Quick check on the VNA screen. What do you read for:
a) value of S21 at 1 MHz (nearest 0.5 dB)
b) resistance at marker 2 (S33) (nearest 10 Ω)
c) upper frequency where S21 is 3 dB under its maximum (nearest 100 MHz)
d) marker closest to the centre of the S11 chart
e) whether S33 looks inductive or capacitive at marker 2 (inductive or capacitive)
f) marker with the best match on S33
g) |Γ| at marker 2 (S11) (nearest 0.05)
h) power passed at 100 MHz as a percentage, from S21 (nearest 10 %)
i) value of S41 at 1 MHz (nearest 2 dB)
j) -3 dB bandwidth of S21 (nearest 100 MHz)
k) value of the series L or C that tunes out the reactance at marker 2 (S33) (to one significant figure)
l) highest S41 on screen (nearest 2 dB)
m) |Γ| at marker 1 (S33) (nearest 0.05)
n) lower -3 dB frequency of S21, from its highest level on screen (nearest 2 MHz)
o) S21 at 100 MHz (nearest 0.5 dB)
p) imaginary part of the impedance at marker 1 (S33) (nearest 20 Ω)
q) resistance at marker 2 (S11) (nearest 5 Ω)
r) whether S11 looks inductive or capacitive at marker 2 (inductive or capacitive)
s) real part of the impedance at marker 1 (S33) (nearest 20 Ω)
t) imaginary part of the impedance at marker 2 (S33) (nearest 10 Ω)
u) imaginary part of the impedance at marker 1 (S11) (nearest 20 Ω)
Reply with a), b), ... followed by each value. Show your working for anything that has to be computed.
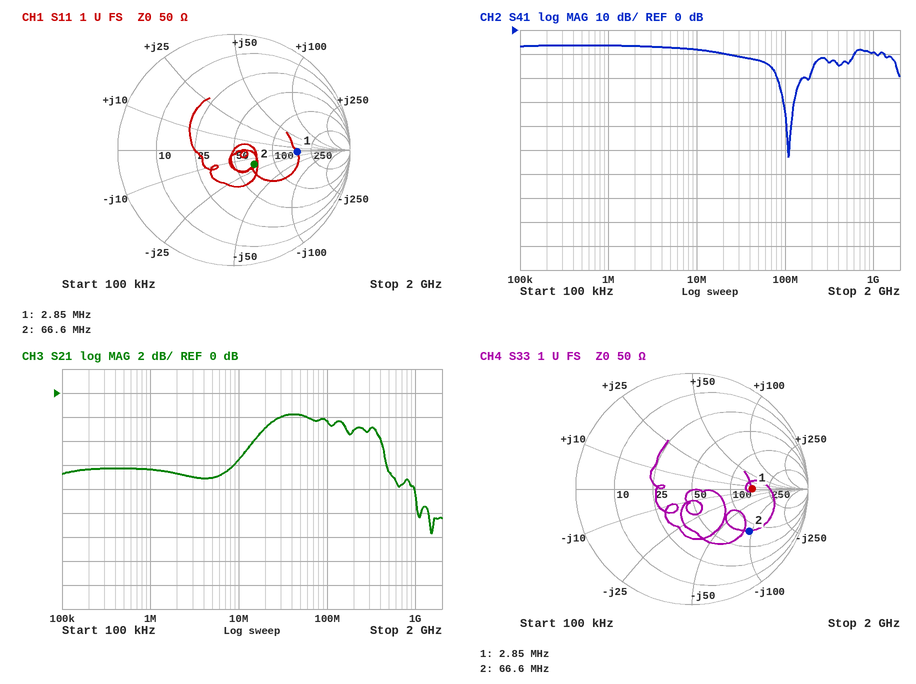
a) -6.5 dB
b) 80 Ω
c) 400 MHz
d) marker 2
e) capacitive
f) marker 1
g) 0.20
h) 10^(-2.5/10) ≈ 56.2 %, so 60 % to the nearest 10 %
i) -6 dB
j) 400 MHz − 12 MHz = 388 MHz
k) L = 90 Ω/(2π × 66.6 MHz) ≈ 215 nH, so 200 nH to one significant figure
l) -6 dB
m) 0.50
n) 12 MHz
o) -2.5 dB
p) 0 Ω
q) 70 Ω
r) capacitive
s) 160 Ω
t) -90 Ω
u) 0 Ω
